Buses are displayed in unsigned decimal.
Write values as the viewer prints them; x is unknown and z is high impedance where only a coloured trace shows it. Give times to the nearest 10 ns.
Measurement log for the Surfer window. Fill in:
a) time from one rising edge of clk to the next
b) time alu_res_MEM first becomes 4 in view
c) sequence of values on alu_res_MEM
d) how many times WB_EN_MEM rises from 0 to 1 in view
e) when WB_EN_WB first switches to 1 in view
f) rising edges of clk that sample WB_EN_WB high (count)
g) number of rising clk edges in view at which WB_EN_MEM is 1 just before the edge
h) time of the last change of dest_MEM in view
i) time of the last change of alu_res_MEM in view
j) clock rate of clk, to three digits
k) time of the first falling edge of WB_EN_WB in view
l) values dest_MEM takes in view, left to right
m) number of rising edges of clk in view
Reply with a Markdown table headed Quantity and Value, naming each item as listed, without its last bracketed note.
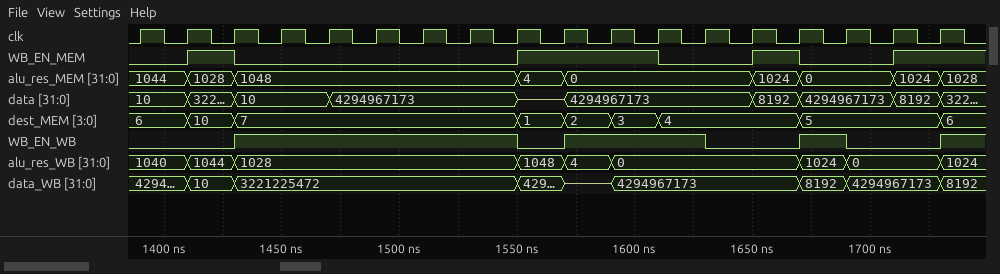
| Quantity | Value |
|---|---|
| time from one rising edge of clk to the next | 20 ns |
| time alu_res_MEM first becomes 4 in view | 1550 ns |
| sequence of values on alu_res_MEM | 1044, 1028, 1048, 4, 0, 1024, 0, 1024, 1028 |
| how many times WB_EN_MEM rises from 0 to 1 in view | 4 |
| when WB_EN_WB first switches to 1 in view | 1430 ns |
| rising edges of clk that sample WB_EN_WB high | 10 |
| number of rising clk edges in view at which WB_EN_MEM is 1 just before the edge | 6 |
| time of the last change of dest_MEM in view | 1730 ns |
| time of the last change of alu_res_MEM in view | 1730 ns |
| clock rate of clk, to three digits | 50.0 MHz |
| time of the first falling edge of WB_EN_WB in view | 1550 ns |
| values dest_MEM takes in view, left to right | 6, 10, 7, 1, 2, 3, 4, 5, 6 |
| number of rising edges of clk in view | 18 |
